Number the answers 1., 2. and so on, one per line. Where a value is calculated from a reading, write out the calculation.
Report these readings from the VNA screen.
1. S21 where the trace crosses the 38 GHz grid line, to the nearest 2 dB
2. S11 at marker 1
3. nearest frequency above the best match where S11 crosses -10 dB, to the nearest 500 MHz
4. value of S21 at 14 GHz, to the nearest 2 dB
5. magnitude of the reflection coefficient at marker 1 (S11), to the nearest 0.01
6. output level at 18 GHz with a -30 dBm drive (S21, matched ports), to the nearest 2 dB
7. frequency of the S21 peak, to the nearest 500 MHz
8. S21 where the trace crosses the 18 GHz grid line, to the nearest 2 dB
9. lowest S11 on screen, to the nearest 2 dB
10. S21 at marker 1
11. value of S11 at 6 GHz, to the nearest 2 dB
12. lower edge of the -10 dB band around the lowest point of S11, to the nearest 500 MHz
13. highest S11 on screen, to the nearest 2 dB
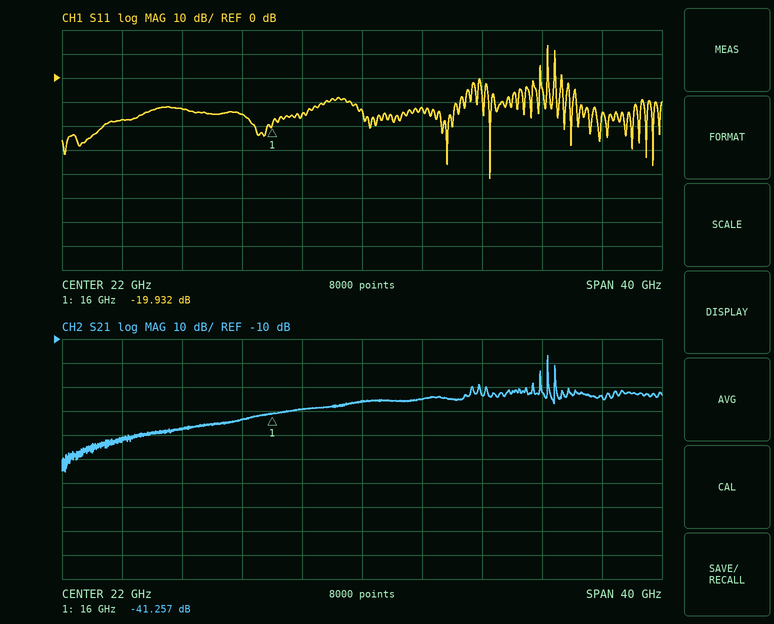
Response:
1. -34 dB
2. -19.932 dB
3. 30.5 GHz
4. -44 dB
5. 10^(-19.932/20) ≈ 0.10
6. -30 dBm + (-40 dB) = -70 dBm
7. 34.5 GHz
8. -40 dB
9. -42 dB
10. -41.257 dB
11. -18 dB
12. 30.5 GHz
13. 14 dB
